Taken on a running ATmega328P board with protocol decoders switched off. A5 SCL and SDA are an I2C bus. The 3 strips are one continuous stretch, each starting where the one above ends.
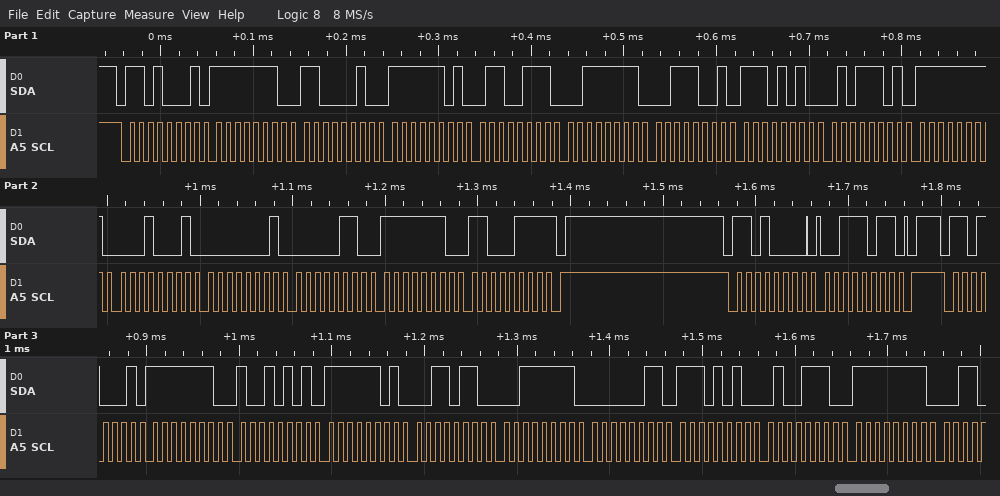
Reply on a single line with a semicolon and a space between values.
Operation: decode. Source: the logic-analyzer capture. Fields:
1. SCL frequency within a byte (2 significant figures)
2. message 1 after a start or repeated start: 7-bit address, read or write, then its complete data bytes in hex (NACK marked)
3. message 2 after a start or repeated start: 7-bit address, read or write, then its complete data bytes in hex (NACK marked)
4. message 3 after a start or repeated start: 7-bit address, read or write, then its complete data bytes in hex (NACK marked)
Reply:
100 kHz; 0x68 read: FE C2 FD 67 3F 39 EA 5D FF 11 01 06 FE C7 NACK; 0x68 write: 3B; 0x68 read: FE 95 FD 36 3F 03 EA 4E FF
